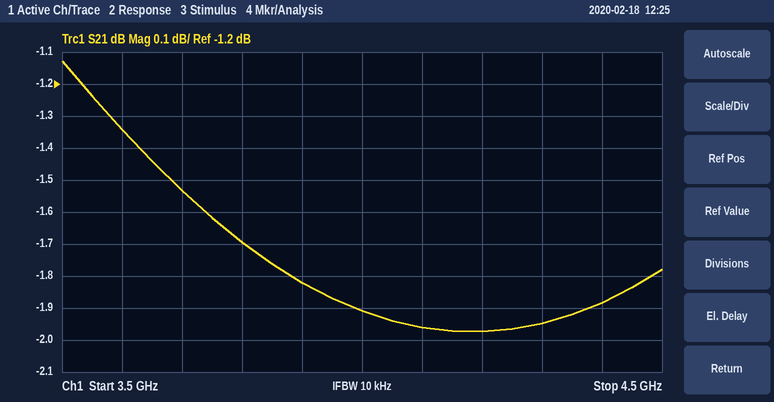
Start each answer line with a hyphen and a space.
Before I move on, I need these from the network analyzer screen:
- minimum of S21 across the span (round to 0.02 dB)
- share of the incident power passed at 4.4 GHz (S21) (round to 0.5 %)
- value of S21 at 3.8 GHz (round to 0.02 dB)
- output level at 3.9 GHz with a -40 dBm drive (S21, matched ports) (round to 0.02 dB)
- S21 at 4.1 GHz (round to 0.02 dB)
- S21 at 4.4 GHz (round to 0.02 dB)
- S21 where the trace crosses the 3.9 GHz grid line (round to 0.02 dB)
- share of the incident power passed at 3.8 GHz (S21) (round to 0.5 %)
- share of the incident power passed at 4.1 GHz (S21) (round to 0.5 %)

- -1.98 dB
- 65.0 %
- -1.70 dB
- -41.82 dBm
- -1.96 dB
- -1.88 dB
- -1.82 dB
- 67.5 %
- 63.5 %
